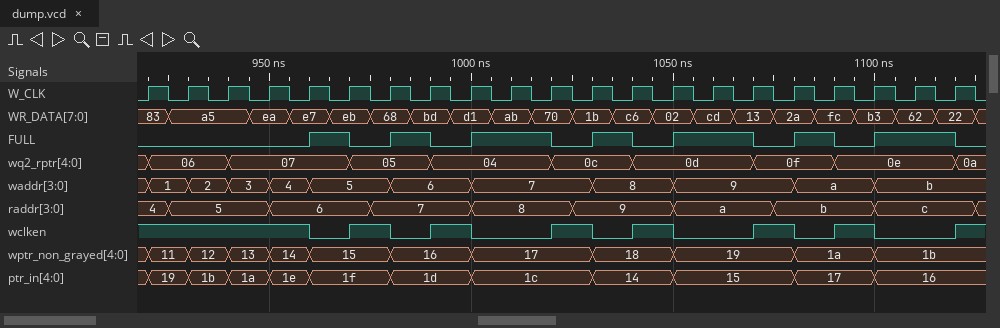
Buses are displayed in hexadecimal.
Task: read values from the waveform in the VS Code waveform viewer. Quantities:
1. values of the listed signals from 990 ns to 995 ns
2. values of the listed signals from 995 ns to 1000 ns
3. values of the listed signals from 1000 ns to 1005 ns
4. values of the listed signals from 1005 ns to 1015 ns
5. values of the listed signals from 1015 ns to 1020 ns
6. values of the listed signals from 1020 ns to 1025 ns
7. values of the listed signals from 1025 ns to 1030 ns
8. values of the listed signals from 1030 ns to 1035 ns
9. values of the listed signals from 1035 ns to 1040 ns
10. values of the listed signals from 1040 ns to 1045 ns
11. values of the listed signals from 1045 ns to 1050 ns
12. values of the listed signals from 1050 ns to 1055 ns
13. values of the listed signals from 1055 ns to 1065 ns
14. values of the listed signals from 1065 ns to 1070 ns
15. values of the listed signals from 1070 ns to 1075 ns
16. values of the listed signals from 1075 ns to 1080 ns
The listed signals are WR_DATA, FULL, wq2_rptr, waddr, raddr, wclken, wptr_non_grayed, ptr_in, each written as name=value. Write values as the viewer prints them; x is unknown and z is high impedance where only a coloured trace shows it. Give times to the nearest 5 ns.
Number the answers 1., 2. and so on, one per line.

1. WR_DATA=bd, FULL=0, wq2_rptr=04, waddr=6, raddr=7, wclken=1, wptr_non_grayed=16, ptr_in=1d
2. WR_DATA=d1, FULL=0, wq2_rptr=04, waddr=6, raddr=7, wclken=1, wptr_non_grayed=16, ptr_in=1d
3. WR_DATA=d1, FULL=1, wq2_rptr=04, waddr=7, raddr=8, wclken=0, wptr_non_grayed=17, ptr_in=1c
4. WR_DATA=ab, FULL=1, wq2_rptr=04, waddr=7, raddr=8, wclken=0, wptr_non_grayed=17, ptr_in=1c
5. WR_DATA=70, FULL=1, wq2_rptr=04, waddr=7, raddr=8, wclken=0, wptr_non_grayed=17, ptr_in=1c
6. WR_DATA=70, FULL=0, wq2_rptr=0c, waddr=7, raddr=8, wclken=1, wptr_non_grayed=17, ptr_in=1c
7. WR_DATA=1b, FULL=0, wq2_rptr=0c, waddr=7, raddr=9, wclken=1, wptr_non_grayed=17, ptr_in=1c
8. WR_DATA=1b, FULL=1, wq2_rptr=0c, waddr=8, raddr=9, wclken=0, wptr_non_grayed=18, ptr_in=14
9. WR_DATA=c6, FULL=1, wq2_rptr=0c, waddr=8, raddr=9, wclken=0, wptr_non_grayed=18, ptr_in=14
10. WR_DATA=c6, FULL=0, wq2_rptr=0d, waddr=8, raddr=9, wclken=1, wptr_non_grayed=18, ptr_in=14
11. WR_DATA=02, FULL=0, wq2_rptr=0d, waddr=8, raddr=9, wclken=1, wptr_non_grayed=18, ptr_in=14
12. WR_DATA=02, FULL=1, wq2_rptr=0d, waddr=9, raddr=a, wclken=0, wptr_non_grayed=19, ptr_in=15
13. WR_DATA=cd, FULL=1, wq2_rptr=0d, waddr=9, raddr=a, wclken=0, wptr_non_grayed=19, ptr_in=15
14. WR_DATA=13, FULL=1, wq2_rptr=0d, waddr=9, raddr=a, wclken=0, wptr_non_grayed=19, ptr_in=15
15. WR_DATA=13, FULL=0, wq2_rptr=0f, waddr=9, raddr=a, wclken=1, wptr_non_grayed=19, ptr_in=15
16. WR_DATA=2a, FULL=0, wq2_rptr=0f, waddr=9, raddr=b, wclken=1, wptr_non_grayed=19, ptr_in=15
